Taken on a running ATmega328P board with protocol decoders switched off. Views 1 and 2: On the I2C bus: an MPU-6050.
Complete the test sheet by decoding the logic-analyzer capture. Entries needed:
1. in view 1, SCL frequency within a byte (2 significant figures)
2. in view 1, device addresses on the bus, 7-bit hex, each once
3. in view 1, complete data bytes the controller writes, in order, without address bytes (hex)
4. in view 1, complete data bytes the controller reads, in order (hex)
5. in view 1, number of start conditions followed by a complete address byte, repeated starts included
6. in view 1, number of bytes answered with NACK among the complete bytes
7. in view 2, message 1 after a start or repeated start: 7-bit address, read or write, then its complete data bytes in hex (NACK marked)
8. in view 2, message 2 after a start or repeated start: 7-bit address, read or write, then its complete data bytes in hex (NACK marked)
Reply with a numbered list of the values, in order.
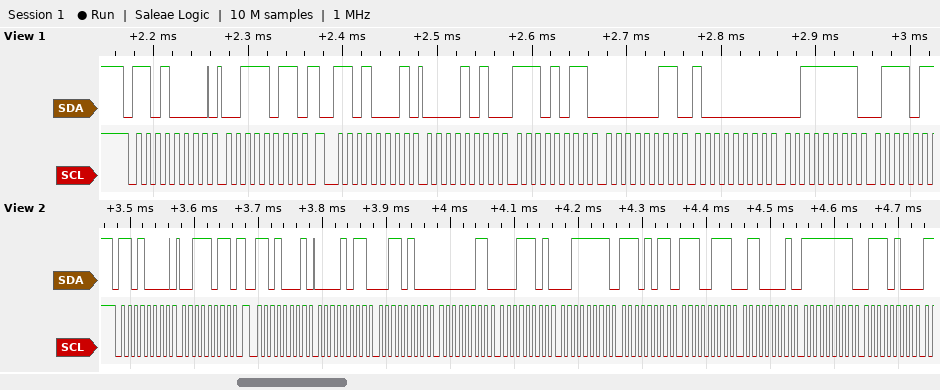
1. 100 kHz
2. 0x68
3. 3B
4. 0A EB 03 80 3F
5. 2
6. 0
7. 0x68 write: 3B
8. 0x68 read: 0B 34 03 1D 3F EB E7 61 FF 74
